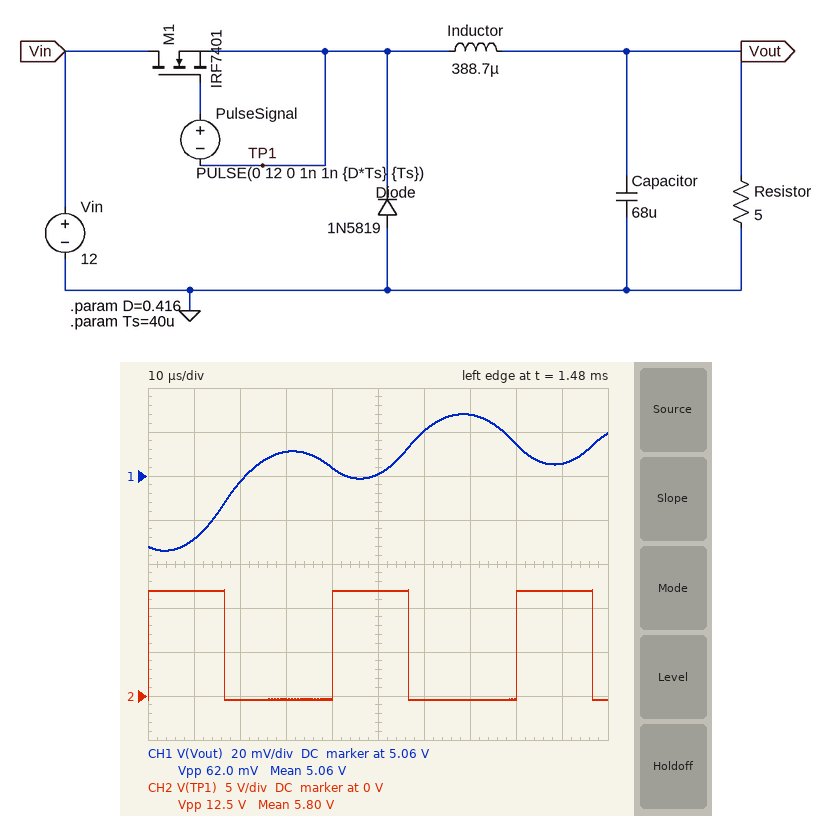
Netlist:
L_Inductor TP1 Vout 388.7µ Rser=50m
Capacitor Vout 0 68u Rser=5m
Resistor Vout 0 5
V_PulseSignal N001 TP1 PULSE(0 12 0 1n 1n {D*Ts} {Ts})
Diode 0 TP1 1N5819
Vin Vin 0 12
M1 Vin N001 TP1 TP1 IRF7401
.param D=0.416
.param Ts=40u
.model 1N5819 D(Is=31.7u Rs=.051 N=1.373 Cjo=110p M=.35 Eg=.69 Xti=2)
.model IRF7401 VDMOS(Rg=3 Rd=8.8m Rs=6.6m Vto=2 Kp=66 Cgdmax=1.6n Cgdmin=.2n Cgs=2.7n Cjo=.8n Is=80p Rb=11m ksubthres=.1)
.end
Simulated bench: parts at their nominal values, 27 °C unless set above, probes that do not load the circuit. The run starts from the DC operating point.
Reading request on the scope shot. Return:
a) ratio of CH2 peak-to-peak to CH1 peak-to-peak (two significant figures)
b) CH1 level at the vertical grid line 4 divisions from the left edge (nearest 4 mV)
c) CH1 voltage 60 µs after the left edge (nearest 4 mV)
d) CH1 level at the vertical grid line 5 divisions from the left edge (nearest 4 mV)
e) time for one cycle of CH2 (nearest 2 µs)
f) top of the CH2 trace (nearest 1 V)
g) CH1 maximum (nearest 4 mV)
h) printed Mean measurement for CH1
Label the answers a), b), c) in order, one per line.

a) 200
b) 5.064 V
c) 5.080 V
d) 5.060 V
e) 40 µs
f) 12 V
g) 5.088 V
h) 5.06 V
